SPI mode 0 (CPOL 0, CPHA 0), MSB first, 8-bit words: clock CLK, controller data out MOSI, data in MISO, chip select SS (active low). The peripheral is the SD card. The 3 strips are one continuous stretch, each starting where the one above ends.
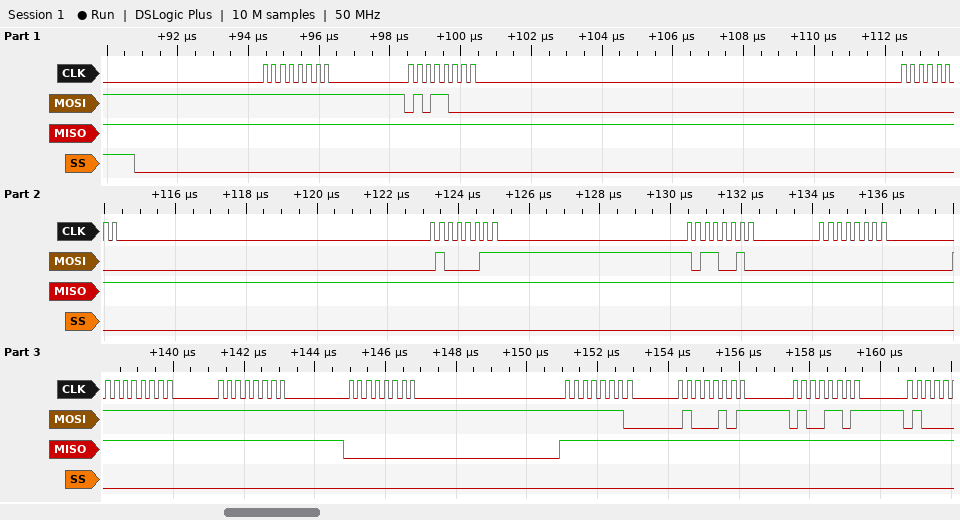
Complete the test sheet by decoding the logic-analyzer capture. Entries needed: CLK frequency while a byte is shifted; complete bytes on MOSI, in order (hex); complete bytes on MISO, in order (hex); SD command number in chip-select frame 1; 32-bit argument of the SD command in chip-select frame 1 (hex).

4 MHz
0xFF 0x58 0x00 0x43 0xB2 0x00 0xFF 0xFF 0xFF 0xFE 0x45 0x4D
0xFF 0xFF 0xFF 0xFF 0xFF 0xFF 0xFF 0xFF 0x00 0xFF 0xFF 0xFF
CMD24
0x0043B200
